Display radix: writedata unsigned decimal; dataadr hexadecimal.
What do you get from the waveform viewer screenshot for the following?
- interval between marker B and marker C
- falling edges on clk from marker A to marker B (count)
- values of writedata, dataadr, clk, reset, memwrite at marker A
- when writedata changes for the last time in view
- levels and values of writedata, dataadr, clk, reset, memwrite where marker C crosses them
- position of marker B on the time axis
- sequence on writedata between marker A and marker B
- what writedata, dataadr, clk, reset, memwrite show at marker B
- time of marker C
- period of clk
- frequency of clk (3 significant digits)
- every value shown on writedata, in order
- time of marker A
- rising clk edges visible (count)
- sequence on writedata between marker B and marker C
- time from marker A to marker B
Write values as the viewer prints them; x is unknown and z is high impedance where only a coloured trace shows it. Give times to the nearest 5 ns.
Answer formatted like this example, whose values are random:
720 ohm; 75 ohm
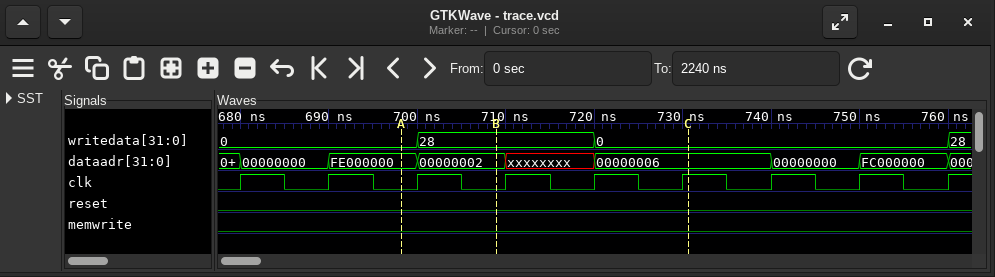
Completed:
20 ns; 1; writedata=0, dataadr=FE000000, clk=0, reset=0, memwrite=0; 760 ns; writedata=0, dataadr=00000006, clk=1, reset=0, memwrite=0; 710 ns; 0, 28; writedata=28, dataadr=00000002, clk=0, reset=0, memwrite=0; 730 ns; 10 ns; 100 MHz; 0, 28, 0, 28; 700 ns; 9; 28, 0; 10 ns
